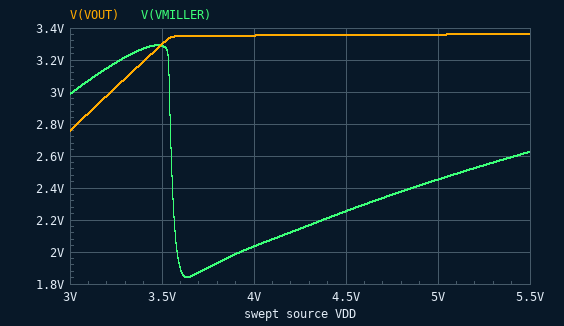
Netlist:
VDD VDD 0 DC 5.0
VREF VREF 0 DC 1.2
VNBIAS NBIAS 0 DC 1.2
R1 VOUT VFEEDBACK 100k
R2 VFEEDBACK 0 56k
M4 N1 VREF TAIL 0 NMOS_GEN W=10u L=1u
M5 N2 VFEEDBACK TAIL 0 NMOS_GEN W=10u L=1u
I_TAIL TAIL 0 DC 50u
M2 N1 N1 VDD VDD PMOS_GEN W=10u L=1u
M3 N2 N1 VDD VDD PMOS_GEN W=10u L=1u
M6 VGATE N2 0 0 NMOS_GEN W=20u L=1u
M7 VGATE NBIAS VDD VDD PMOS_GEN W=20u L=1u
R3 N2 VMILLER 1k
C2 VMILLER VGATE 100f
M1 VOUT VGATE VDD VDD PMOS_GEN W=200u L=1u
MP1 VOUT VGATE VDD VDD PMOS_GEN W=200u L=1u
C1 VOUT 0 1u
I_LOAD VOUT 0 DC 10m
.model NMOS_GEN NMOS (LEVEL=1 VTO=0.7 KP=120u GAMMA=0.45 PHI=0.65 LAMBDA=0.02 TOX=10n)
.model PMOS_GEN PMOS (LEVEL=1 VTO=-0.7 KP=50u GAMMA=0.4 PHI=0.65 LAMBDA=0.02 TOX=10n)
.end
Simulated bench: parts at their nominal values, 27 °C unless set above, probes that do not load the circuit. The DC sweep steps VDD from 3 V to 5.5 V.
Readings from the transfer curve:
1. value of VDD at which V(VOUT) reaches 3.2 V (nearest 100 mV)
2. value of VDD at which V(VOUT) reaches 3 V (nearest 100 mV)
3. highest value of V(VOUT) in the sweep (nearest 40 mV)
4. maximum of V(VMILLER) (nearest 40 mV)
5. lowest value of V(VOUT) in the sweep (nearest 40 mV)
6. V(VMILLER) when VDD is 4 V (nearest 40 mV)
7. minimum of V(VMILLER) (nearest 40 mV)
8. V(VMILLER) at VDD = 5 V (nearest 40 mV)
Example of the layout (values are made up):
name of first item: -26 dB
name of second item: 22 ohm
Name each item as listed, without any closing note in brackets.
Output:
value of VDD at which V(VOUT) reaches 3.2 V: 3.4 V
value of VDD at which V(VOUT) reaches 3 V: 3.2 V
highest value of V(VOUT) in the sweep: 3.36 V
maximum of V(VMILLER): 3.28 V
lowest value of V(VOUT) in the sweep: 2.76 V
V(VMILLER) when VDD is 4 V: 2.04 V
minimum of V(VMILLER): 1.84 V
V(VMILLER) at VDD = 5 V: 2.44 V
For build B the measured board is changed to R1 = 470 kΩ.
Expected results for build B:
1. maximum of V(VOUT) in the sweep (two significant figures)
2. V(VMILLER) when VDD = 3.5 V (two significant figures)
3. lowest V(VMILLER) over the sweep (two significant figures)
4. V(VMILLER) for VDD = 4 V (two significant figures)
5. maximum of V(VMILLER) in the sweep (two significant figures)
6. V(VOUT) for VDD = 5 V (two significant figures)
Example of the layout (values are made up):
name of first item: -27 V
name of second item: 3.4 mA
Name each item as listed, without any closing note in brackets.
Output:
maximum of V(VOUT) in the sweep: 5.4 V
V(VMILLER) when VDD = 3.5 V: 3.5 V
lowest V(VMILLER) over the sweep: 3.0 V
V(VMILLER) for VDD = 4 V: 4.0 V
maximum of V(VMILLER) in the sweep: 5.5 V
V(VOUT) for VDD = 5 V: 4.9 V
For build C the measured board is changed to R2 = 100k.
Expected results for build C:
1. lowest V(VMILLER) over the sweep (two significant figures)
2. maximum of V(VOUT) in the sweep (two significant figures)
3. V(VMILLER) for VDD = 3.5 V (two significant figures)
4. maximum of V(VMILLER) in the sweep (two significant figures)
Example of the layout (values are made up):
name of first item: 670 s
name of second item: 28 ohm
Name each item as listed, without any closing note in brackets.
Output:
lowest V(VMILLER) over the sweep: 1.4 V
maximum of V(VOUT) in the sweep: 2.4 V
V(VMILLER) for VDD = 3.5 V: 1.7 V
maximum of V(VMILLER) in the sweep: 2.6 V
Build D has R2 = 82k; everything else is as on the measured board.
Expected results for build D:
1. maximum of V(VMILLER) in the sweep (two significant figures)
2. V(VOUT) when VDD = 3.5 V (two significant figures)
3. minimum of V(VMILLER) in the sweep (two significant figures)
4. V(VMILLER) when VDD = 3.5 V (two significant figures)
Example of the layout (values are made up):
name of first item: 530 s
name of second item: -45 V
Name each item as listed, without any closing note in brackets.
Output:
maximum of V(VMILLER) in the sweep: 2.6 V
V(VOUT) when VDD = 3.5 V: 2.7 V
minimum of V(VMILLER) in the sweep: 1.4 V
V(VMILLER) when VDD = 3.5 V: 1.7 V
